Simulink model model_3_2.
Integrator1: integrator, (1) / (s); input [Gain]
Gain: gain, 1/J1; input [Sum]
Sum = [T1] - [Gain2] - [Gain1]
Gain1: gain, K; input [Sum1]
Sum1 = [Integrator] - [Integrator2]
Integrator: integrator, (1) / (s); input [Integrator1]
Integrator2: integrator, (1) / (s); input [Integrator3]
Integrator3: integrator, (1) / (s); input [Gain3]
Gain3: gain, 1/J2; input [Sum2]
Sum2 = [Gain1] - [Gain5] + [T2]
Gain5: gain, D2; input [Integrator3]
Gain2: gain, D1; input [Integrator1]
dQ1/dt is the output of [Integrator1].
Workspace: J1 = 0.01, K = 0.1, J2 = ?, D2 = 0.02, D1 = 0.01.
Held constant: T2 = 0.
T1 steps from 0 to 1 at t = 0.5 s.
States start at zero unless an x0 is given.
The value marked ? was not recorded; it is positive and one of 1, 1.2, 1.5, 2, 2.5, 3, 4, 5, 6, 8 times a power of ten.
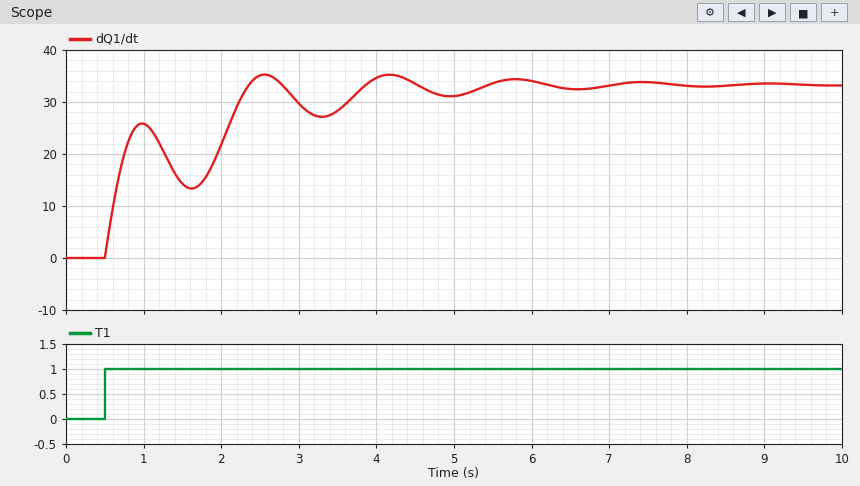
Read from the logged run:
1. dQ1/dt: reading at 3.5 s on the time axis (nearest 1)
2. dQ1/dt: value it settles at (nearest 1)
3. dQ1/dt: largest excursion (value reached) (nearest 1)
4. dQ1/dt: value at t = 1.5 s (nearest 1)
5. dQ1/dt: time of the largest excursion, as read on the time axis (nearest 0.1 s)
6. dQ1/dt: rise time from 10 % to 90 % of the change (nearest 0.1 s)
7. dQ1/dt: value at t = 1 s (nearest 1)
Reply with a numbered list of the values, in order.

1. 28
2. 33
3. 35
4. 14
5. 2.6 s
6. 1.7 s
7. 26
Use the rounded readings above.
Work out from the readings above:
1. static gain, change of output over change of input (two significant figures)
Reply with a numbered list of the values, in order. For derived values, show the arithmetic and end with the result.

1. (33 - 0) / (1 - 0) = 33
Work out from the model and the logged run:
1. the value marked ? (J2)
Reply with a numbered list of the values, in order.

1. 0.02
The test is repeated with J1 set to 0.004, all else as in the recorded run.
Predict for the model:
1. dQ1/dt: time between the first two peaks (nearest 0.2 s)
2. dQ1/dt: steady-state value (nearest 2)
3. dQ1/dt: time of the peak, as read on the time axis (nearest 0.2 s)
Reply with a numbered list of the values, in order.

1. 1.2 s
2. 34
3. 0.8 s
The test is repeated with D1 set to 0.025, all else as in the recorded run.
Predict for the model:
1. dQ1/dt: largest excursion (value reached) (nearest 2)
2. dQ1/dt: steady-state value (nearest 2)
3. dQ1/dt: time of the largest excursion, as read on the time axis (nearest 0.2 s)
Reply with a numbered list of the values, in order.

1. 24
2. 22
3. 2.6 s
